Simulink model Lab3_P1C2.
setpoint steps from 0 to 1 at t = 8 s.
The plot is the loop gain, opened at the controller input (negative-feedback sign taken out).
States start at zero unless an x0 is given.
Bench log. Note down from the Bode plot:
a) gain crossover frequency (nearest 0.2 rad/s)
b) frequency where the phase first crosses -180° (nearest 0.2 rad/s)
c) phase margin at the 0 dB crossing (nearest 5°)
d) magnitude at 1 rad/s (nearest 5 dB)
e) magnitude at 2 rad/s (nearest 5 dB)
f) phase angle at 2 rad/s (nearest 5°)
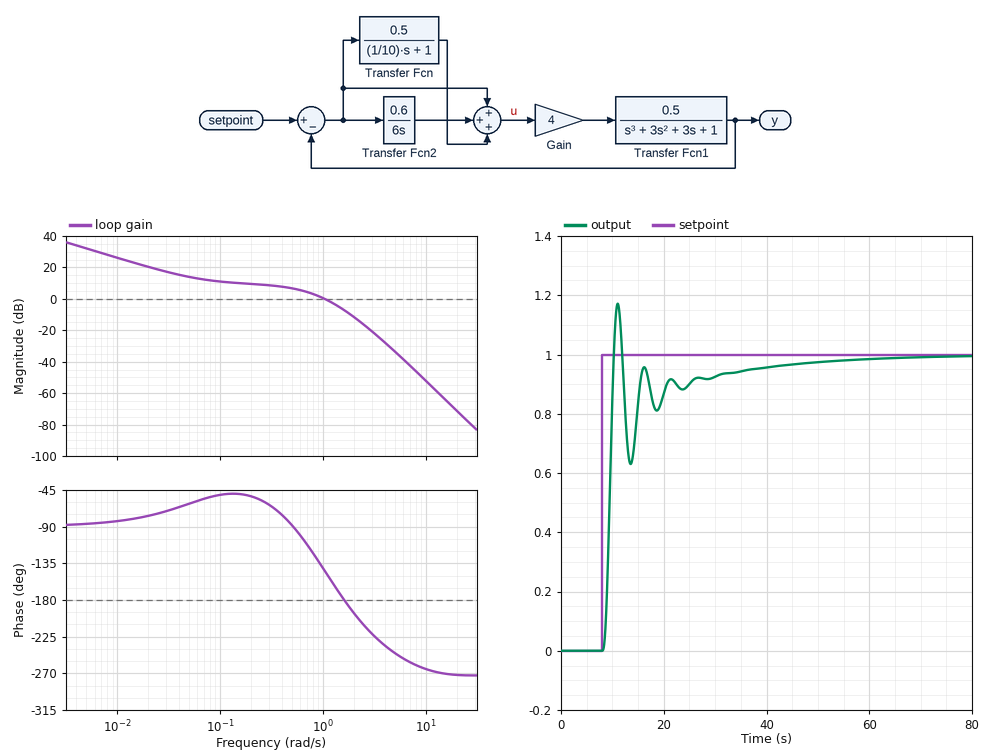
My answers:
1.0 rad/s
1.6 rad/s
35°
0 dB
-10 dB
-195°
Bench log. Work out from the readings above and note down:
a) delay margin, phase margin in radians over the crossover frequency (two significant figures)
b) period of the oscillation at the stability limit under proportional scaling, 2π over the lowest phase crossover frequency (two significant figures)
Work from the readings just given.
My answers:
0.61 s
3.9 s
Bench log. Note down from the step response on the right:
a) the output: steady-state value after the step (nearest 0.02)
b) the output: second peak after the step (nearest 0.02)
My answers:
1.00
0.96
